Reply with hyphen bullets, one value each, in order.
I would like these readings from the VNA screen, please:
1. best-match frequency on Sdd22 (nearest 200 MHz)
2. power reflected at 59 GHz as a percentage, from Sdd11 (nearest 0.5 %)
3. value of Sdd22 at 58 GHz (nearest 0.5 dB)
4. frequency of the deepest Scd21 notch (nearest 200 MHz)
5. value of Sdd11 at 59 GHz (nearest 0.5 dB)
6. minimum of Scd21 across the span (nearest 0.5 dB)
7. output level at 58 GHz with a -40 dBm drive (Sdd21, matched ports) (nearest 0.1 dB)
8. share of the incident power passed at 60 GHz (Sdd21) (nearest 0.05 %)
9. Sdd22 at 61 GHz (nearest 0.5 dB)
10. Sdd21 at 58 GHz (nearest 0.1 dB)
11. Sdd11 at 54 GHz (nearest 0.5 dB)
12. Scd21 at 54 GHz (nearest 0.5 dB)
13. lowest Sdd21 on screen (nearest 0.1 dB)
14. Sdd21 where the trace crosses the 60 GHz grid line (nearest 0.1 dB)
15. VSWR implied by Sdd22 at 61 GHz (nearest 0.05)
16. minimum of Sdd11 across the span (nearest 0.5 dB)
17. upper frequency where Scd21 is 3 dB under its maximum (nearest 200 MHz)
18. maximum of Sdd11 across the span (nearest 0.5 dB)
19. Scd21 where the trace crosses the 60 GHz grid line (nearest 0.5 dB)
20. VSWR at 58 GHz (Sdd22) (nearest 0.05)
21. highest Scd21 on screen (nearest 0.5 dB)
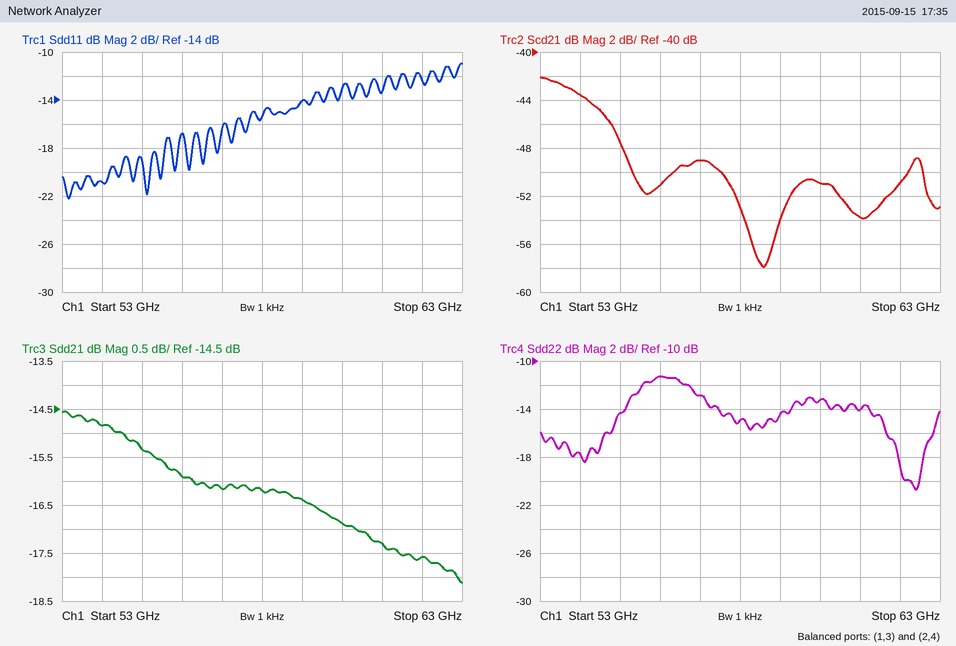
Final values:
- 62.4 GHz
- 4.0 %
- -15.0 dB
- 58.6 GHz
- -14.0 dB
- -58.0 dB
- -56.2 dBm
- 2.05 %
- -14.0 dB
- -16.2 dB
- -21.0 dB
- -43.5 dB
- -18.1 dB
- -16.9 dB
- 1.50
- -22.0 dB
- 54.6 GHz
- -11.0 dB
- -51.0 dB
- 1.45
- -42.0 dB
